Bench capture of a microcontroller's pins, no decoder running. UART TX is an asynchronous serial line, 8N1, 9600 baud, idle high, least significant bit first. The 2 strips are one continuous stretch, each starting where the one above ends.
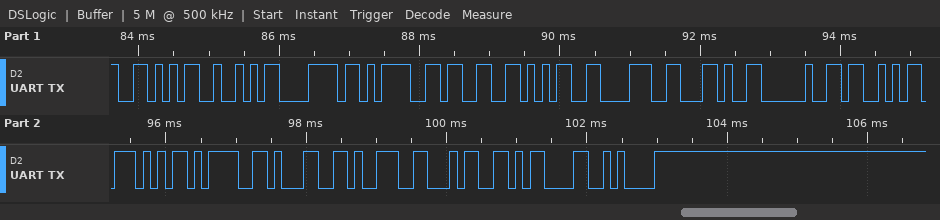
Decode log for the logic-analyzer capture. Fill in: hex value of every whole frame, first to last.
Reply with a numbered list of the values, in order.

1. 0x56 0x52 0x78 0x3D 0x33 0x35 0x38 0x2C 0x20 0x53 0x57 0x3D 0x31 0x39 0x34 0x0D 0x0A
